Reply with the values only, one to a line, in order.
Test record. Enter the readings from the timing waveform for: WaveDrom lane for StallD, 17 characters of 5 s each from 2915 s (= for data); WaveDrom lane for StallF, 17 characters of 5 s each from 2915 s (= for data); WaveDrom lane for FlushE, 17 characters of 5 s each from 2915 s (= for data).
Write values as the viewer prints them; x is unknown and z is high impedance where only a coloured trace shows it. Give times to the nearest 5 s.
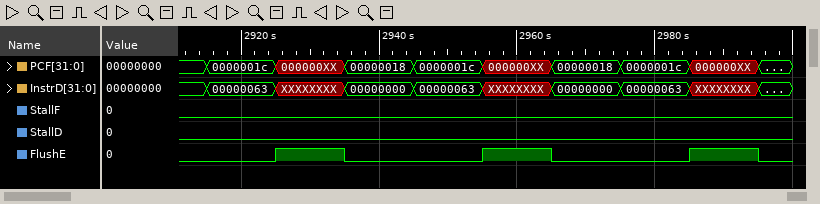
{name: 'StallD', wave: '0................'}
{name: 'StallF', wave: '0................'}
{name: 'FlushE', wave: '0.1.0...1.0...1.0'}
